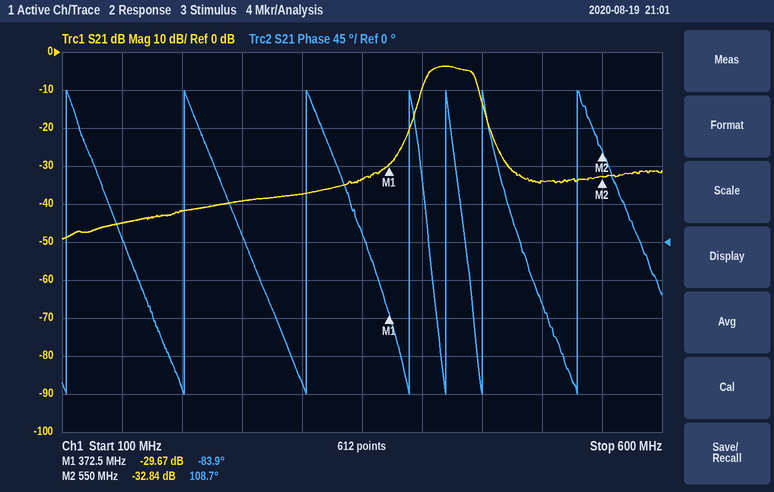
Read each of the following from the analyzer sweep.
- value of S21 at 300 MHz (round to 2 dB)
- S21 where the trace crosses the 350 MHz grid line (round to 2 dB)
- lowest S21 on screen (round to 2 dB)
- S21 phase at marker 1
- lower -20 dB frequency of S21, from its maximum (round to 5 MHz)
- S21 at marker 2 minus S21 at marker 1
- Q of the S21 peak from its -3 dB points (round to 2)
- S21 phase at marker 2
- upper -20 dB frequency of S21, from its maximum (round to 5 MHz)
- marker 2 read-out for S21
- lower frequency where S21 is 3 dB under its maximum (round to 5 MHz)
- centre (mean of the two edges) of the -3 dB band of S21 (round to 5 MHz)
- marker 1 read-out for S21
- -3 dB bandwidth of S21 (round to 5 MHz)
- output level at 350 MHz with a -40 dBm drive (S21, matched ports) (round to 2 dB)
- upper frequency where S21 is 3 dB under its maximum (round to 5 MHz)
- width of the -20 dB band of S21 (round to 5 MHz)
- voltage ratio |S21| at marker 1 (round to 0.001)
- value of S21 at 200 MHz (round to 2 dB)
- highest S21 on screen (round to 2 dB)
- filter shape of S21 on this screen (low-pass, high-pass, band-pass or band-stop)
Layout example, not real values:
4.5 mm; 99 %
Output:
-38 dB; -34 dB; -50 dB; -83.9°; 385 MHz; -3.17 dB; 10; 108.7°; 460 MHz; -32.84 dB; 405 MHz; 425 MHz; -29.67 dB; 40 MHz; -74 dBm; 445 MHz; 75 MHz; 0.033; -42 dB; -4 dB; band-pass
